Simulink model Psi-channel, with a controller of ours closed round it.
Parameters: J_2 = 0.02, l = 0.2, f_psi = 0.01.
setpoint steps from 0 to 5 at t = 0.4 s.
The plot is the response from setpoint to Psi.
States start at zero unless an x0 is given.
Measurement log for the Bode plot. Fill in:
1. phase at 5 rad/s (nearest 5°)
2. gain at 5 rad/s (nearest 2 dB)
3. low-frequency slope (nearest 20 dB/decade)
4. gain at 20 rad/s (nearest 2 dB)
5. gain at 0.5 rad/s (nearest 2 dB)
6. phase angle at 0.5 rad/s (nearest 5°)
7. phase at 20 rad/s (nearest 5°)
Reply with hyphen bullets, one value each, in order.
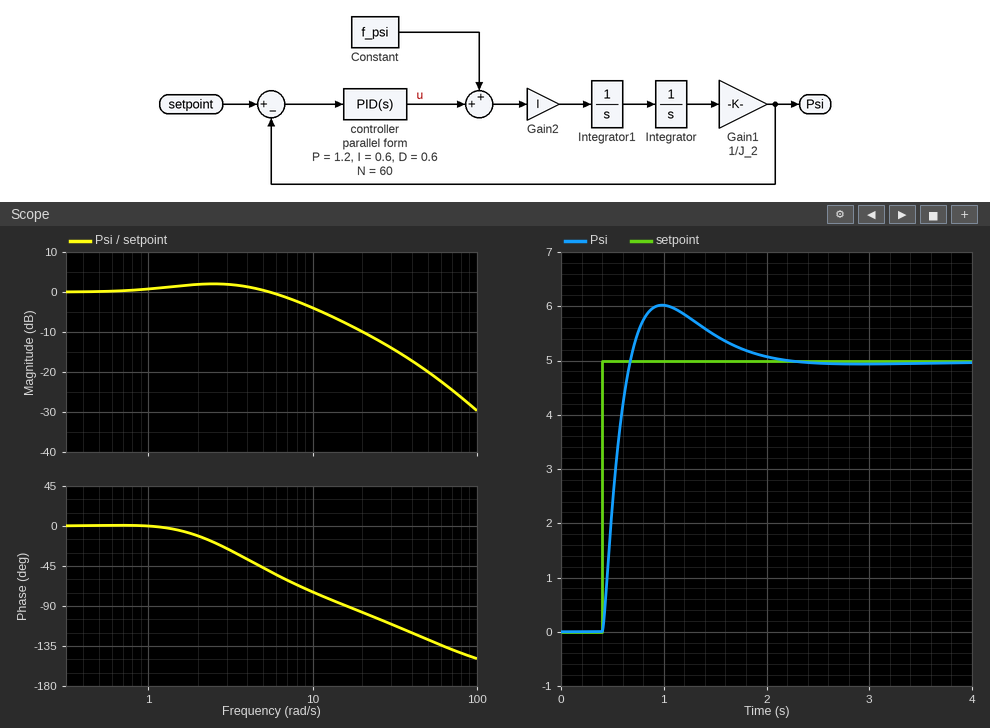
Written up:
- -45°
- 0 dB
- 0 dB/decade
- -10 dB
- 0 dB
- 0°
- -95°
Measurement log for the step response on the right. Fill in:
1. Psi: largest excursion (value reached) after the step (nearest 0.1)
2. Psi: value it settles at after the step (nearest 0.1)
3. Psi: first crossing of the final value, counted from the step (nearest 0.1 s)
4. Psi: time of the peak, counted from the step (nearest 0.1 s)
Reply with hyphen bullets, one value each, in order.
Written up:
- 6.0
- 5.0
- 0.3 s
- 0.6 s
